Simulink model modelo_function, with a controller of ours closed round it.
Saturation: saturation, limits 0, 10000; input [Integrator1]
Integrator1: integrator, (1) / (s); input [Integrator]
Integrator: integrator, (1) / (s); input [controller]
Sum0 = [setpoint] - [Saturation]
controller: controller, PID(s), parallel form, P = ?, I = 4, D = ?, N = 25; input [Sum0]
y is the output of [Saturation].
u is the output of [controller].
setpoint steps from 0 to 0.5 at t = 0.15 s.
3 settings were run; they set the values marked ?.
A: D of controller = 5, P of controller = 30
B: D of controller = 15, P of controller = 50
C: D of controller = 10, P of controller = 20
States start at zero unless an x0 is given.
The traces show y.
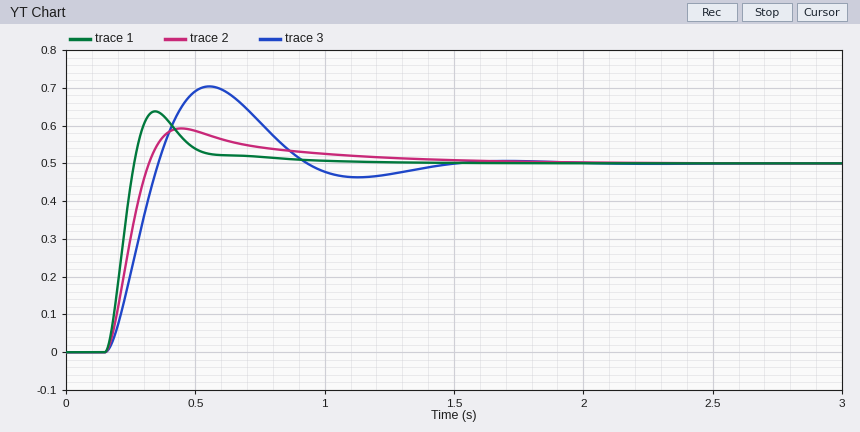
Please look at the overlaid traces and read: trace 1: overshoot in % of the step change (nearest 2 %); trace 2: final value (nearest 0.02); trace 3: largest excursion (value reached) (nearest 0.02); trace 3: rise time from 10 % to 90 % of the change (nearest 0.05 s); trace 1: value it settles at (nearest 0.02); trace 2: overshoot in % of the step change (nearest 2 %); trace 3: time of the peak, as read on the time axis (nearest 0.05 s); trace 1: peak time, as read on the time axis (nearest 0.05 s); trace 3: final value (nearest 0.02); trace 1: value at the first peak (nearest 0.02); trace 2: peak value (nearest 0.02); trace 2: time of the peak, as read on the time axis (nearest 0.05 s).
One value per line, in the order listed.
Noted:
28 %
0.50
0.70
0.15 s
0.50
18 %
0.55 s
0.35 s
0.50
0.64
0.60
0.45 s
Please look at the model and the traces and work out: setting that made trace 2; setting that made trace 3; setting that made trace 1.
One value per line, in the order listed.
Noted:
C
A
B
